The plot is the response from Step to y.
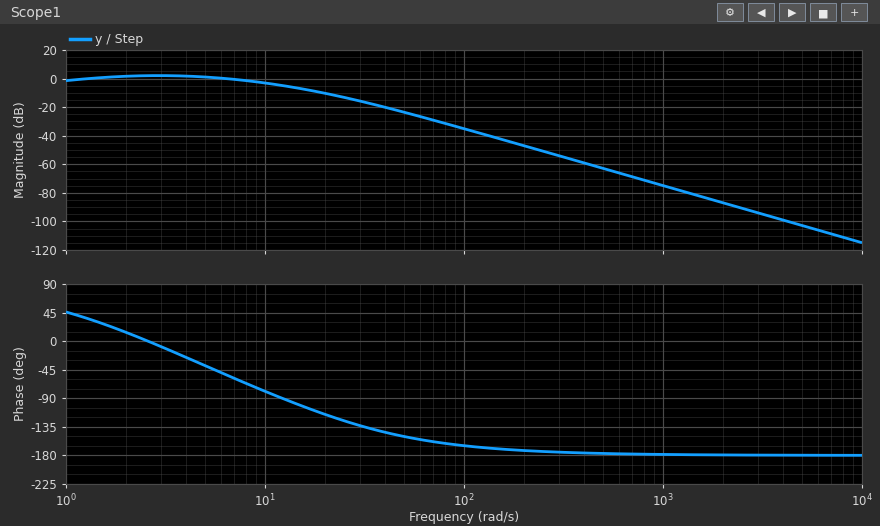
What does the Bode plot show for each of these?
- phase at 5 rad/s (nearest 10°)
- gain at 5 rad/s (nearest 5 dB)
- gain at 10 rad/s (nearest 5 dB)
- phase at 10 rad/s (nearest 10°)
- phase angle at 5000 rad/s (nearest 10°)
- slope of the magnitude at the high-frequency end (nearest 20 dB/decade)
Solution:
-40°
0 dB
-5 dB
-80°
-180°
-40 dB/decade
